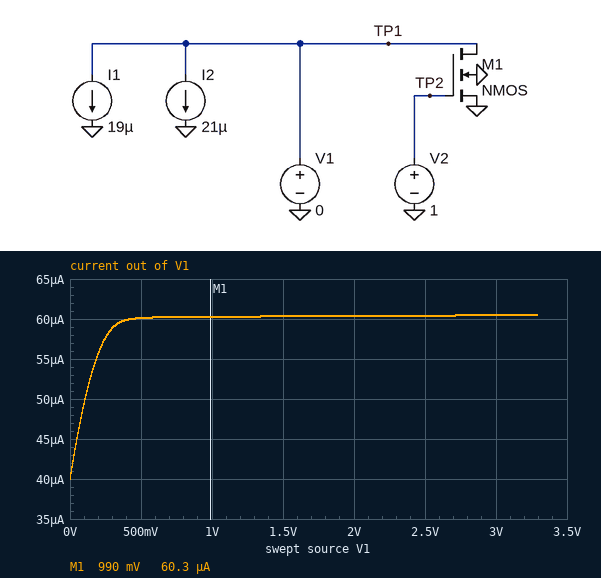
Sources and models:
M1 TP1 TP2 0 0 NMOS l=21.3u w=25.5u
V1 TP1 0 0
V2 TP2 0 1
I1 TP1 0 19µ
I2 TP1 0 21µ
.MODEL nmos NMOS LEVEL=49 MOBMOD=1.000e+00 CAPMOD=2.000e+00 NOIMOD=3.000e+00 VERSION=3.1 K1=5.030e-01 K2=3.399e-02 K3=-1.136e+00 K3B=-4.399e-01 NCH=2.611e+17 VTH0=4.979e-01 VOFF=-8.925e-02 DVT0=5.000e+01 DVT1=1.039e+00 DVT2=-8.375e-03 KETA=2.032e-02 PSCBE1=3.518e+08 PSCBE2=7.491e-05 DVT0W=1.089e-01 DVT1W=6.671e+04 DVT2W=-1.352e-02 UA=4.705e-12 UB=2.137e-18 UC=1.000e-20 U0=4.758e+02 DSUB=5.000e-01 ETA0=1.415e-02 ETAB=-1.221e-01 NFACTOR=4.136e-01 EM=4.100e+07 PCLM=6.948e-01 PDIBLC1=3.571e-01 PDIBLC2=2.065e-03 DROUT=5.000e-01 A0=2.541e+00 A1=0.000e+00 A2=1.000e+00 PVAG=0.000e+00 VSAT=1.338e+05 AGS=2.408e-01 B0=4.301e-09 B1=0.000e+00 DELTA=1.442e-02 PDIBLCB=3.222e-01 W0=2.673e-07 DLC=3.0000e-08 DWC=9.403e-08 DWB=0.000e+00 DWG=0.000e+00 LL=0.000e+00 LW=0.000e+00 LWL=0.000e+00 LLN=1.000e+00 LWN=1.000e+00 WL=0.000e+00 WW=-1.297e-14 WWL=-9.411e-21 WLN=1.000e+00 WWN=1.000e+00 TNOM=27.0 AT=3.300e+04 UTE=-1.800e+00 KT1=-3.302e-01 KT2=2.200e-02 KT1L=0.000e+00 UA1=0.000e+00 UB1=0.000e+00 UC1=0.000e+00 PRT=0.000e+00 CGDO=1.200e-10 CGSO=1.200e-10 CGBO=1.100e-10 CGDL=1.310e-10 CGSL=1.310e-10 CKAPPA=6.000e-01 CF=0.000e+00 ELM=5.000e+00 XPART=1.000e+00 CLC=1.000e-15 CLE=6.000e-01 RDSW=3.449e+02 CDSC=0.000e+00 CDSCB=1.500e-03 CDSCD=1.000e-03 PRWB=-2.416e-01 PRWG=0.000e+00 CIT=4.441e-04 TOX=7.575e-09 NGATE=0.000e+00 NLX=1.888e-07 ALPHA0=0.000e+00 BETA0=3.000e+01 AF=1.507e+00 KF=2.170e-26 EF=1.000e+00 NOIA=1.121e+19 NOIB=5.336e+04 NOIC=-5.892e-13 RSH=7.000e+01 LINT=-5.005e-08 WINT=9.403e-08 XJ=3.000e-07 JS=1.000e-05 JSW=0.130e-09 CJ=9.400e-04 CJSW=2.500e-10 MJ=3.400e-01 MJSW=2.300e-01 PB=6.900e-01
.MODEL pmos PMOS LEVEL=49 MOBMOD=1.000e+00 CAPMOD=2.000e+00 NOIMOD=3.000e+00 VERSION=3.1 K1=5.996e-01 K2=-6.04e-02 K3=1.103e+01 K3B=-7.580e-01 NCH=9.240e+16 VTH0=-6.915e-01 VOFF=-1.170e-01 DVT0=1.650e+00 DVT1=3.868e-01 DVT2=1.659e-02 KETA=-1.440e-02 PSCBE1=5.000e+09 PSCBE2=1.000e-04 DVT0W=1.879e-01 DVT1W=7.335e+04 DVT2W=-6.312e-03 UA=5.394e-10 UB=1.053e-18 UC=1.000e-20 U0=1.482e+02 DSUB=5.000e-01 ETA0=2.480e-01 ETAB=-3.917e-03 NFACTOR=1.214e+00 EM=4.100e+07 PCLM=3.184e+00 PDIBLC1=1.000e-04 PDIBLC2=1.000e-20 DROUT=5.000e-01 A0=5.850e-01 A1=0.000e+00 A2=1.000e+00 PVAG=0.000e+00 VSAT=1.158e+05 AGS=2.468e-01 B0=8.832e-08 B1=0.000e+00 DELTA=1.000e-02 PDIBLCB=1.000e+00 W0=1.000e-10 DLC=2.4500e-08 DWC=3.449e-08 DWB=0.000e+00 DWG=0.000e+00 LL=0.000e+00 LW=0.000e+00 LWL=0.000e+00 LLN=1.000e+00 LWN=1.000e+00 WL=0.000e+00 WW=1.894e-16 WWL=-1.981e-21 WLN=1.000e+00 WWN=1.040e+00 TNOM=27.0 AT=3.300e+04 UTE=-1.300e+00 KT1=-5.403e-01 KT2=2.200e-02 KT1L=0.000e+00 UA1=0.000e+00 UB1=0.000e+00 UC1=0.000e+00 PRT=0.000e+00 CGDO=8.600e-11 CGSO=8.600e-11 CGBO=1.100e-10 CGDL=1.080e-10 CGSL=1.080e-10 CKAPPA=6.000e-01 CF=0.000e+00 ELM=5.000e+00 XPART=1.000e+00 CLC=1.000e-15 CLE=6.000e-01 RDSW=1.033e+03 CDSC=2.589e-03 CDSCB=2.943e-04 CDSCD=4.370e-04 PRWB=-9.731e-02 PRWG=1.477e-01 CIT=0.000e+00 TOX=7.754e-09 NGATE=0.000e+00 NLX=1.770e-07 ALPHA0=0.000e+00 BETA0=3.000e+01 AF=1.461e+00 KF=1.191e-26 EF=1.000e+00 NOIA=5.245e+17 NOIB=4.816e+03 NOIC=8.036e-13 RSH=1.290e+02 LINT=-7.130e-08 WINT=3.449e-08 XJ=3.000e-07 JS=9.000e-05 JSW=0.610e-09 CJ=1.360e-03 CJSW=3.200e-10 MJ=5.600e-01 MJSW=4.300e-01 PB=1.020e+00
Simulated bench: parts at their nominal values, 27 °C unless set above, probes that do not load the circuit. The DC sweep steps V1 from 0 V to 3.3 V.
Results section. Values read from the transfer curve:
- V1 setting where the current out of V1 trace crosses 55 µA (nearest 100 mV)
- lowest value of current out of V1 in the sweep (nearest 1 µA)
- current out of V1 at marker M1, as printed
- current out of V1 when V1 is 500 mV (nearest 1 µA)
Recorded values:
200 mV
40 µA
60.3 µA
60 µA
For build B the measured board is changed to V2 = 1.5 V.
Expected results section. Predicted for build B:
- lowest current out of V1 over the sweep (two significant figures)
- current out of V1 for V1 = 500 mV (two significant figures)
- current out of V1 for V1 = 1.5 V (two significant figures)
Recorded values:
40 µA
110 µA
120 µA
